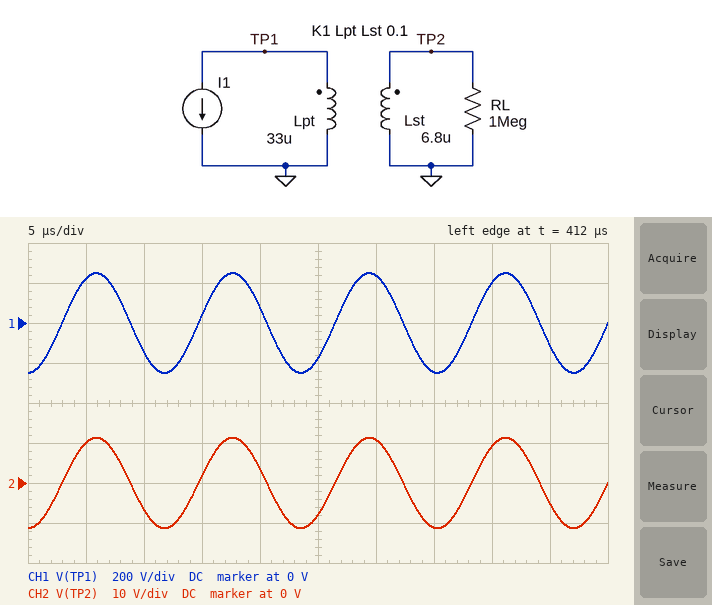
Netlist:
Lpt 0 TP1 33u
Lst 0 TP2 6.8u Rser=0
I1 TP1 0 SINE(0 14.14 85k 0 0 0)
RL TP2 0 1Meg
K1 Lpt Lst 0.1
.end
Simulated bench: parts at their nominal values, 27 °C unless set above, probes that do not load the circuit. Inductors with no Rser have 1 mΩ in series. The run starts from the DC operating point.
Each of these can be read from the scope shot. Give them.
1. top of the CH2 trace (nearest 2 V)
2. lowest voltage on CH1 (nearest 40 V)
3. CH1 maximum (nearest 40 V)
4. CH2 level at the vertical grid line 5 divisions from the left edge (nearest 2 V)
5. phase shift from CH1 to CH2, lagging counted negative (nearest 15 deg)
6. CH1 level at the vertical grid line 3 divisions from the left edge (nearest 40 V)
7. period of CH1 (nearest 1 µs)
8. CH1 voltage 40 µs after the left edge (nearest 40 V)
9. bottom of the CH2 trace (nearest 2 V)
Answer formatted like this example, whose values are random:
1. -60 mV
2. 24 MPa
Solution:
1. 12 V
2. -240 V
3. 240 V
4. -8 V
5. 0 deg
6. 40 V
7. 12 µs
8. 200 V
9. -12 V
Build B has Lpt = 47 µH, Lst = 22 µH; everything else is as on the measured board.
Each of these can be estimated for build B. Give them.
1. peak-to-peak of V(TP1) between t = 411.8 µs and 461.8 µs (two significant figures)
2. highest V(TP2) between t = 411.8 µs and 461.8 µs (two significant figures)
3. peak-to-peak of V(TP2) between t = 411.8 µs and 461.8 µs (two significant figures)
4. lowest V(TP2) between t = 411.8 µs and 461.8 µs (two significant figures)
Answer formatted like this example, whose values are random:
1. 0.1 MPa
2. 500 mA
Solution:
1. 710 V
2. 24 V
3. 49 V
4. -24 V
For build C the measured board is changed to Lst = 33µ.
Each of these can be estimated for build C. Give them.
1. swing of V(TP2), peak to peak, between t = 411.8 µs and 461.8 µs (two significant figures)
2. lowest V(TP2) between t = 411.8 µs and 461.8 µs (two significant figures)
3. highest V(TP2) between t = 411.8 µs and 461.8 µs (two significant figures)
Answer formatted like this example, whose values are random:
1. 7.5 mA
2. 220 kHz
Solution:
1. 50 V
2. -25 V
3. 25 V
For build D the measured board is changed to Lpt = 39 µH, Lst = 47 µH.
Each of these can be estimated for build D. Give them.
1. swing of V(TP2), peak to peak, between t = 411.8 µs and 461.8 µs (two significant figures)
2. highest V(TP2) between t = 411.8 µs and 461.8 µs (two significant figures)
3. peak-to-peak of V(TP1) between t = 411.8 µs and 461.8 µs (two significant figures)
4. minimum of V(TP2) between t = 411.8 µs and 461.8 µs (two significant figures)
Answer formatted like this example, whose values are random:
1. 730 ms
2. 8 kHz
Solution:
1. 65 V
2. 32 V
3. 590 V
4. -32 V
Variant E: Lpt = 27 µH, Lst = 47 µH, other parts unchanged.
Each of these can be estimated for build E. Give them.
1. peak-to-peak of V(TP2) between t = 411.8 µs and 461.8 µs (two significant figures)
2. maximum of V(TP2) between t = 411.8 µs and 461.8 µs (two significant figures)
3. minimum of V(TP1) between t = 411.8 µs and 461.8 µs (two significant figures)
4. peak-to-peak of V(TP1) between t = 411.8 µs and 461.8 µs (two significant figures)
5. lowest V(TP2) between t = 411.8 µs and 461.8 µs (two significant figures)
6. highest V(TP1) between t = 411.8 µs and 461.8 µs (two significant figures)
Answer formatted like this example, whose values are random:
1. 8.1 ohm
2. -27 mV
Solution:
1. 54 V
2. 27 V
3. -200 V
4. 410 V
5. -27 V
6. 200 V
